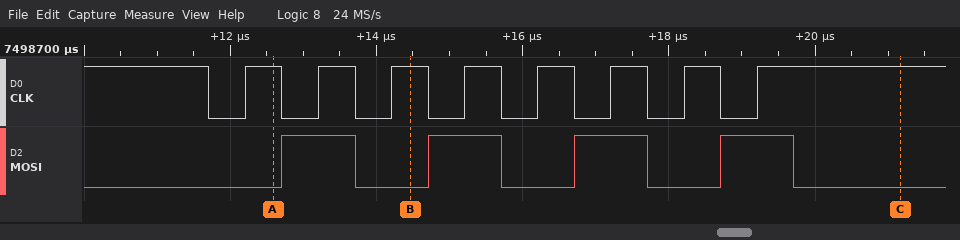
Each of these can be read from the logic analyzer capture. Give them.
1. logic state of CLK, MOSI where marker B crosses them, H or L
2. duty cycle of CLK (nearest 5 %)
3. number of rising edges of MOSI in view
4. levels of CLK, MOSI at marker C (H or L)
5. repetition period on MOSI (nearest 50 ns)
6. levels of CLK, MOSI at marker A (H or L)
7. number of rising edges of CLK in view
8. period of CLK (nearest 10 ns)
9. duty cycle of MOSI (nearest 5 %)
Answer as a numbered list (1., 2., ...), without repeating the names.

1. CLK=H, MOSI=L
2. 50 %
3. 4
4. CLK=H, MOSI=L
5. 2000 ns
6. CLK=H, MOSI=L
7. 8
8. 1000 ns
9. 50 %
